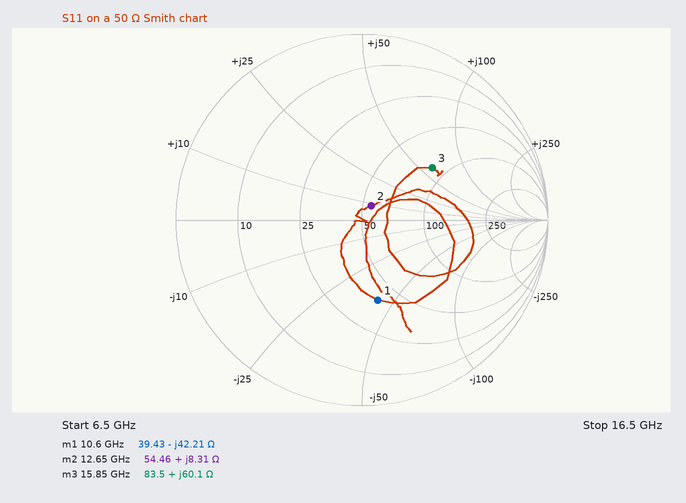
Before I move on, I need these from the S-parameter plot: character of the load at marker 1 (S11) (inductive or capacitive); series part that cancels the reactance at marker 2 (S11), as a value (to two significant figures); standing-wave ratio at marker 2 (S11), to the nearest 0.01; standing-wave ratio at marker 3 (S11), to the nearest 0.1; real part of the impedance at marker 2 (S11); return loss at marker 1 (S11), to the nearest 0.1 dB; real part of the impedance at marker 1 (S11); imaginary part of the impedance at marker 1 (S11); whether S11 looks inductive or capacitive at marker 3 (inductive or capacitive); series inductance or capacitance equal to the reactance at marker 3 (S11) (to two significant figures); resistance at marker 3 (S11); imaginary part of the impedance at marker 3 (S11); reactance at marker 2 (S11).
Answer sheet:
capacitive
1.5 pF
1.20
2.8
54.46 Ω
7.1 dB
39.43 Ω
-42.21 Ω
inductive
600 pH
83.5 Ω
+60.1 Ω
+8.31 Ω
